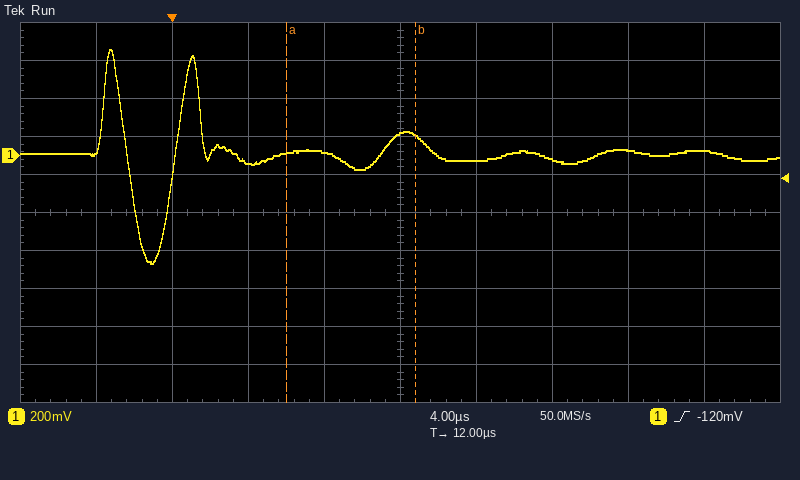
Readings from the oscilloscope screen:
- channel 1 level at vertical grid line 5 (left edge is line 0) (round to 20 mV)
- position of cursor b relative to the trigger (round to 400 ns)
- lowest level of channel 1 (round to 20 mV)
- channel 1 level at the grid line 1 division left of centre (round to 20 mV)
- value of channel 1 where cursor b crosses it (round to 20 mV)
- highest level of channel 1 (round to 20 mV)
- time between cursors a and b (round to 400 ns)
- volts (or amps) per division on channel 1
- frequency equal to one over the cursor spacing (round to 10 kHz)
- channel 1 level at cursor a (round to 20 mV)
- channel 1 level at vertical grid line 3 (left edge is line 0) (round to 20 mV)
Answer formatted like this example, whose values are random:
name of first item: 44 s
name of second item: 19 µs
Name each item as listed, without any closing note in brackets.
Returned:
channel 1 level at vertical grid line 5 (left edge is line 0): 120 mV
position of cursor b relative to the trigger: +12.8 µs
lowest level of channel 1: -560 mV
channel 1 level at the grid line 1 division left of centre: 20 mV
value of channel 1 where cursor b crosses it: 100 mV
highest level of channel 1: 560 mV
time between cursors a and b: 6.8 µs
volts (or amps) per division on channel 1: 200 mV
frequency equal to one over the cursor spacing: 150 kHz
channel 1 level at cursor a: 20 mV
channel 1 level at vertical grid line 3 (left edge is line 0): -40 mV
